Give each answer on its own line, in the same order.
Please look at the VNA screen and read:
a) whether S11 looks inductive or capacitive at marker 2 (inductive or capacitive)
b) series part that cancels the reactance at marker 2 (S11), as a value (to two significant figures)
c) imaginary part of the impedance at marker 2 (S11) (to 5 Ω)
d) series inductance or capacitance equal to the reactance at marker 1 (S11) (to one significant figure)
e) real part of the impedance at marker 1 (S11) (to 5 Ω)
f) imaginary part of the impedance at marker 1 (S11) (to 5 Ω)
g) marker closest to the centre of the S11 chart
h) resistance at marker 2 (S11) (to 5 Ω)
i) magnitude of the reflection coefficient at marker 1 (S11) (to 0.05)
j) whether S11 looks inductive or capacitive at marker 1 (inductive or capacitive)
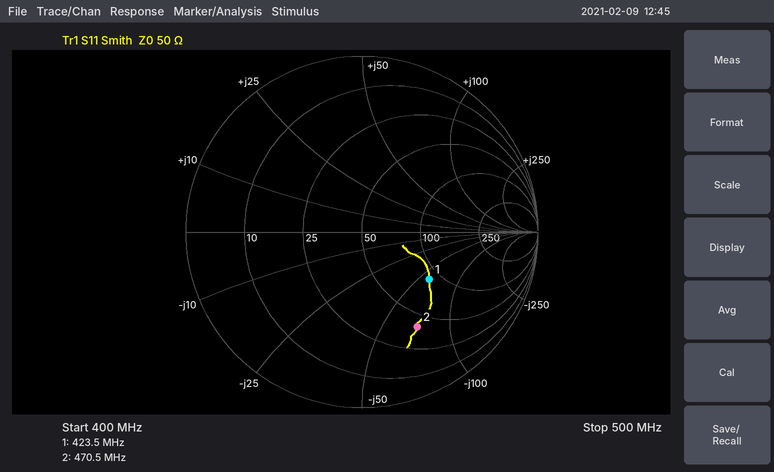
capacitive
24 nH
-70 Ω
6 pF
85 Ω
-60 Ω
marker 1
40 Ω
0.45
capacitive
